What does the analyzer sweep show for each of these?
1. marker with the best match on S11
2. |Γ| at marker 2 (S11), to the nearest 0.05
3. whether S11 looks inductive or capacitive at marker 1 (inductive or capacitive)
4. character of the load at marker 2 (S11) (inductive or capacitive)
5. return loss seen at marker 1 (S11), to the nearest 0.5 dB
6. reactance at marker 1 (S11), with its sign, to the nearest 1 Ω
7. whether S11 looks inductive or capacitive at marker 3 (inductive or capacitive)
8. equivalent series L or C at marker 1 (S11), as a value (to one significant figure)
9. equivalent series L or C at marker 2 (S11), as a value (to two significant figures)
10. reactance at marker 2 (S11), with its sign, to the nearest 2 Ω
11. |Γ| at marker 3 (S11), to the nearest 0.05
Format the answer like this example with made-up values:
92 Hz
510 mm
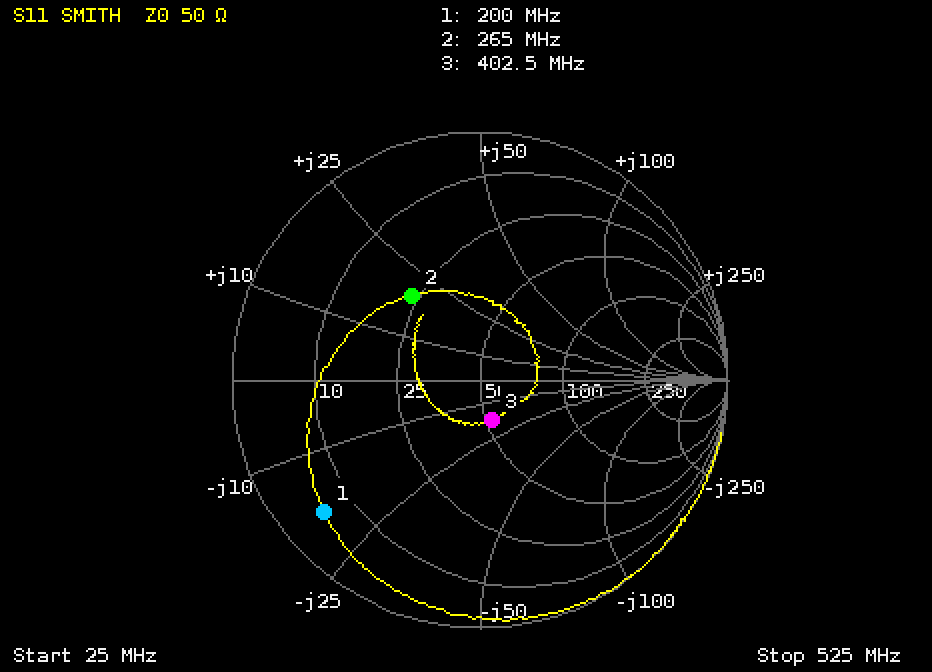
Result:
marker 3
0.45
capacitive
inductive
1.5 dB
-18 Ω
capacitive
40 pF
12 nH
+20 Ω
0.15
